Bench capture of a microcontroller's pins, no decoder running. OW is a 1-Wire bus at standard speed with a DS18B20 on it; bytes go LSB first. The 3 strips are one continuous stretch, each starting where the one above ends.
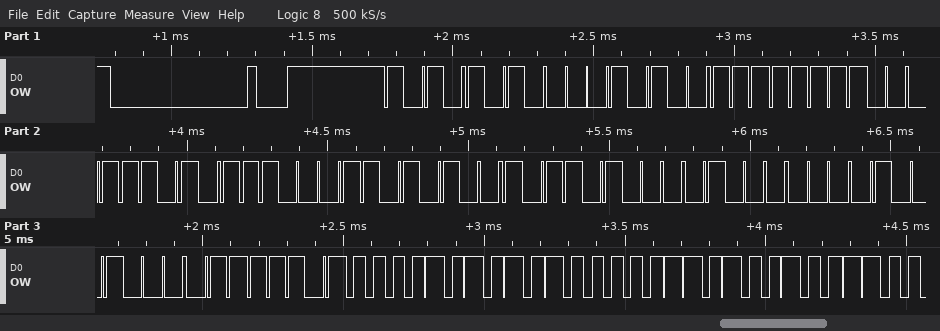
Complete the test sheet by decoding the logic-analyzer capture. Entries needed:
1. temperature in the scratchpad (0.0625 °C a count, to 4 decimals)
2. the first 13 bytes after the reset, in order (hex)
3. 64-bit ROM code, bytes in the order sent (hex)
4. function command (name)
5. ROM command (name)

85.0000 °C
55 28 FF B8 8E 95 16 02 12 BE 50 05 4B
28 FF B8 8E 95 16 02 12
Read Scratchpad
Match ROM
